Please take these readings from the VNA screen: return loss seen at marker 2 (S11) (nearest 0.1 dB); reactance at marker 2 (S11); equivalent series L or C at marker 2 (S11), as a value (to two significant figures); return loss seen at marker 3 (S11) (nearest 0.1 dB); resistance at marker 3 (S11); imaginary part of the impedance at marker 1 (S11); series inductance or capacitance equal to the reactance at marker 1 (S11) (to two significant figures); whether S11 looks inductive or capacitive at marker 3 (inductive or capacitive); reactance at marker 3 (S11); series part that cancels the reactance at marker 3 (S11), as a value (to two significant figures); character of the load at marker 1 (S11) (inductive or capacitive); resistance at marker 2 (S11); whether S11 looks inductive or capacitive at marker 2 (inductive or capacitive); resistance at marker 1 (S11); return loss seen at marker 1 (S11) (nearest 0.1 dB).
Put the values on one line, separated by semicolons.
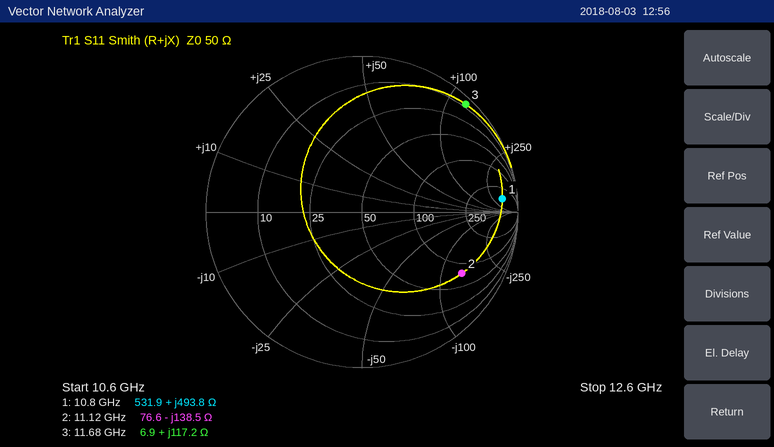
2.5 dB; -138.5 Ω; 100 fF; 0.4 dB; 6.9 Ω; +493.8 Ω; 7.3 nH; inductive; +117.2 Ω; 120 fF; inductive; 76.6 Ω; capacitive; 531.9 Ω; 0.9 dB
